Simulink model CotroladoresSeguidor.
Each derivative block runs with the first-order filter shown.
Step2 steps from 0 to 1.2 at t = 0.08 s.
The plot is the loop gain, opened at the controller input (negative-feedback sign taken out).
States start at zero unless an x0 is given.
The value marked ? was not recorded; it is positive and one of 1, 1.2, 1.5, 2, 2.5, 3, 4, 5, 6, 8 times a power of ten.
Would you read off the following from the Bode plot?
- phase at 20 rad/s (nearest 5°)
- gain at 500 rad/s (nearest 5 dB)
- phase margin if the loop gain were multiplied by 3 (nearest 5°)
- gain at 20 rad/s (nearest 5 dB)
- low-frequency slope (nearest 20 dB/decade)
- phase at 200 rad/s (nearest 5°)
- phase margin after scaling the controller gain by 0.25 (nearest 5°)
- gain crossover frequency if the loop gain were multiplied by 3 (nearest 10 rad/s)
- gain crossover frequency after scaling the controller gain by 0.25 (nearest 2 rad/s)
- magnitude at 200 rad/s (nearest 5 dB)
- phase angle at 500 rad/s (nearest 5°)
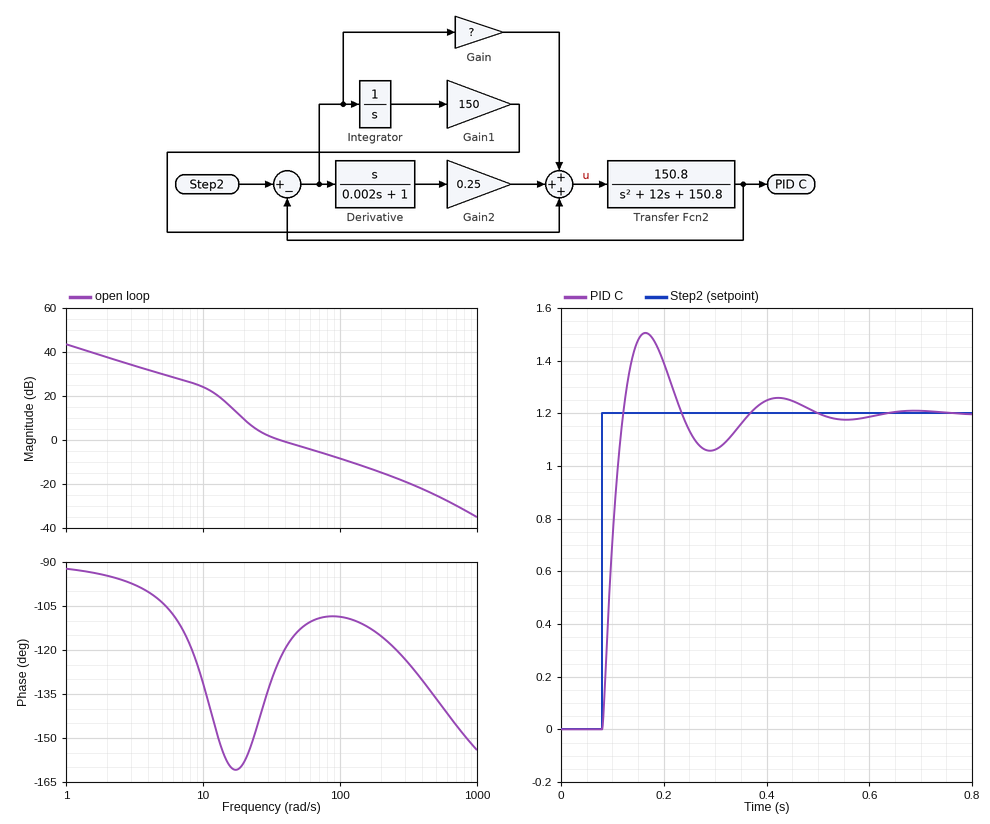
-160°
-25 dB
70°
10 dB
-20 dB/decade
-115°
20°
110 rad/s
18 rad/s
-15 dB
-135°
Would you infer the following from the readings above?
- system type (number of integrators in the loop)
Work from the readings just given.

1
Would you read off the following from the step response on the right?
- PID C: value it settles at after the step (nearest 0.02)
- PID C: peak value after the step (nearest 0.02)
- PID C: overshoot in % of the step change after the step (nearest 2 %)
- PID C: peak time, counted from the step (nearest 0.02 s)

1.20
1.50
26 %
0.08 s
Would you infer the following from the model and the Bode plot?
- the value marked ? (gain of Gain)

6
